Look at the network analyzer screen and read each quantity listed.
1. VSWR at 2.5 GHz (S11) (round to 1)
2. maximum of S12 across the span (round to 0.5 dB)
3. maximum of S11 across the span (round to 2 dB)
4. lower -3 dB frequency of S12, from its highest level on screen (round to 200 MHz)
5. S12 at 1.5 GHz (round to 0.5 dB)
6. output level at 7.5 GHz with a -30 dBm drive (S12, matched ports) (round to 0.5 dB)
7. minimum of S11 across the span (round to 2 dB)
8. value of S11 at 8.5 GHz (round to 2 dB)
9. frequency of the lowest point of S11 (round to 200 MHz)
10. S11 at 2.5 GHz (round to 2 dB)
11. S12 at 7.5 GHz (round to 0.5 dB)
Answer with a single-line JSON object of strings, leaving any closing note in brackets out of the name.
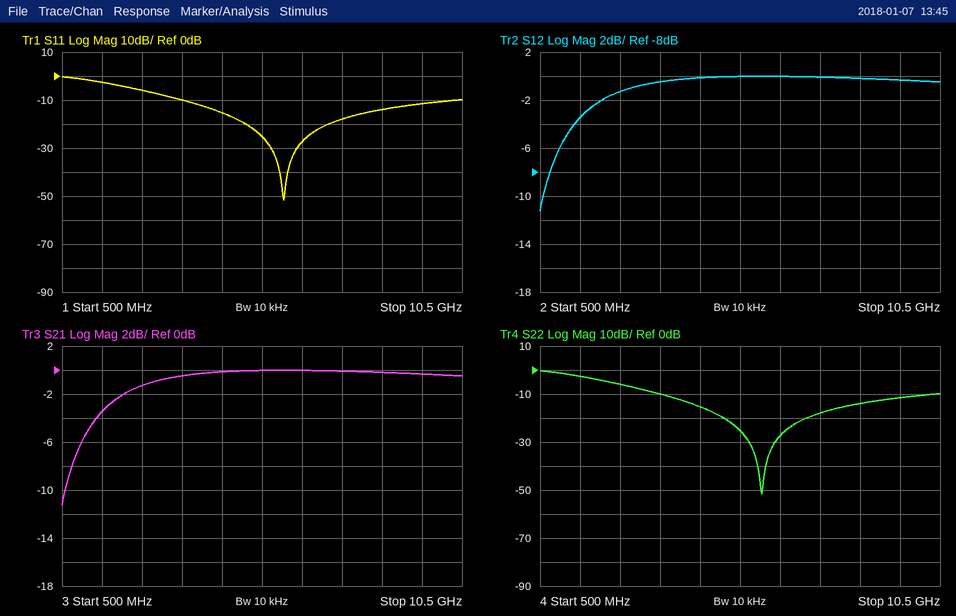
{"VSWR at 2.5 GHz (S11)": "3", "maximum of S12 across the span": "0.0 dB", "maximum of S11 across the span": "0 dB", "lower -3 dB frequency of S12, from its highest level on screen": "1.6 GHz", "S12 at 1.5 GHz": "-3.5 dB", "output level at 7.5 GHz with a -30 dBm drive (S12, matched ports)": "-30.0 dBm", "minimum of S11 across the span": "-52 dB", "value of S11 at 8.5 GHz": "-14 dB", "frequency of the lowest point of S11": "6.0 GHz", "S11 at 2.5 GHz": "-6 dB", "S12 at 7.5 GHz": "0.0 dB"}
